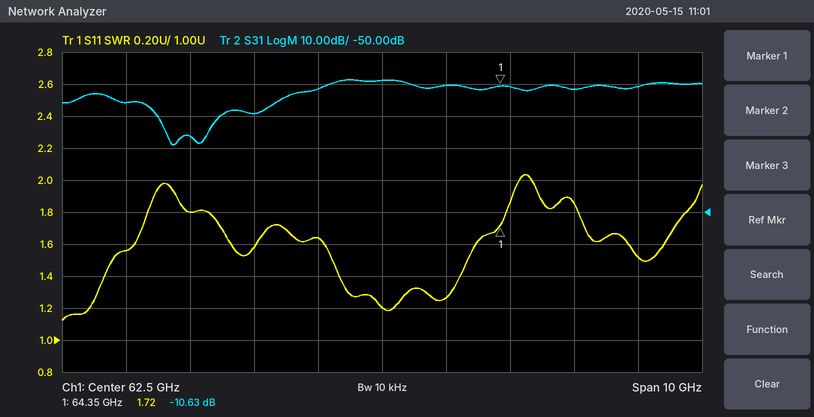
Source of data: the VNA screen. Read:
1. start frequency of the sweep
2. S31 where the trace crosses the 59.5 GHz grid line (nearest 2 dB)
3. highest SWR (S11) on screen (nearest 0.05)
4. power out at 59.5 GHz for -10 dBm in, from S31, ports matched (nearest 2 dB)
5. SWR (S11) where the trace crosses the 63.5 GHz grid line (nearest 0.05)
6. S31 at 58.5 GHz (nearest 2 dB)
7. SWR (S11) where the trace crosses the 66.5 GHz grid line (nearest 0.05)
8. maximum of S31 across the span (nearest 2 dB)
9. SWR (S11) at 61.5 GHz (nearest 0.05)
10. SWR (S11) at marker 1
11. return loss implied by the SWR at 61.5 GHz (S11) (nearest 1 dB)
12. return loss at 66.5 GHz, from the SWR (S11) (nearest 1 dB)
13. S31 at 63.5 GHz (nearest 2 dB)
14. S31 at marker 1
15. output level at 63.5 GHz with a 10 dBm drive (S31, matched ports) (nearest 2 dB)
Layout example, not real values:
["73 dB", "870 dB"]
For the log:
["57.5 GHz", "-26 dB", "2.05", "-36 dBm", "1.25", "-16 dB", "1.50", "-8 dB", "1.65", "1.72", "12 dB", "14 dB", "-10 dB", "-10.63 dB", "0 dBm"]
